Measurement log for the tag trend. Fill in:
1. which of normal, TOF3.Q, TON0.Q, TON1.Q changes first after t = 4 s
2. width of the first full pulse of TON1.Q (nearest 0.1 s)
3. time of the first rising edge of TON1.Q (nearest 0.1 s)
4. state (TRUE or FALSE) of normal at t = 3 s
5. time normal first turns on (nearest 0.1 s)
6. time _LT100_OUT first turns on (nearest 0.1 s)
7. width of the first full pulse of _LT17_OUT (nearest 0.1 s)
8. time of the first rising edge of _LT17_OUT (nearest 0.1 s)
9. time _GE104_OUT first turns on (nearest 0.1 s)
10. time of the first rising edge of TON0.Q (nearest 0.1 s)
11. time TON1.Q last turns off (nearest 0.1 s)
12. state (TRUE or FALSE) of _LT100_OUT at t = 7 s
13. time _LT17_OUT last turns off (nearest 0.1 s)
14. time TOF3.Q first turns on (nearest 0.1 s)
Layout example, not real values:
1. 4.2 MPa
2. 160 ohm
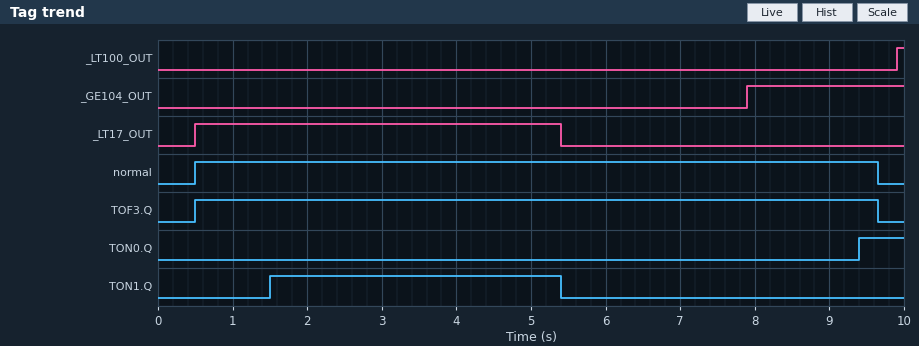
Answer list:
1. TON1.Q
2. 3.9 s
3. 1.5 s
4. TRUE
5. 0.5 s
6. 9.9 s
7. 4.9 s
8. 0.5 s
9. 7.9 s
10. 9.4 s
11. 5.4 s
12. FALSE
13. 5.4 s
14. 0.5 s
